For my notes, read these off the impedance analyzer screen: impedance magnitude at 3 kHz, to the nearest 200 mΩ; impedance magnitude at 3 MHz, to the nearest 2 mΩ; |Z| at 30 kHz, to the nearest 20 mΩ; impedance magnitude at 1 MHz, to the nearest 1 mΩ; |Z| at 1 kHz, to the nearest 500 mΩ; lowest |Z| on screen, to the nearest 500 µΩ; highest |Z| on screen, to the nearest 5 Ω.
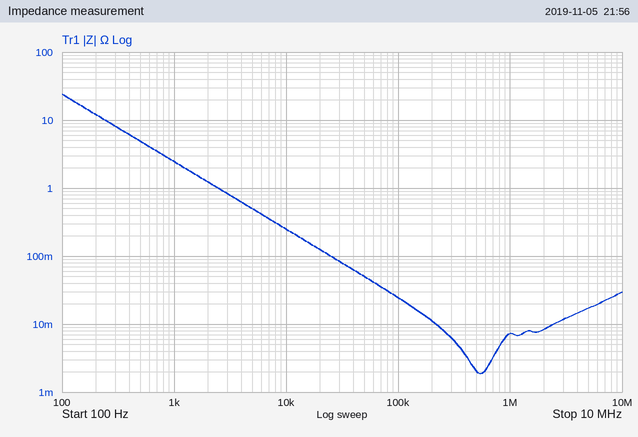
800 mΩ
12 mΩ
80 mΩ
7 mΩ
2.5 Ω
2.0 mΩ
25 Ω
